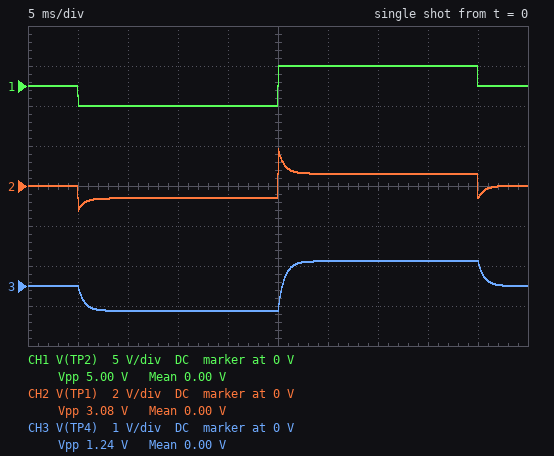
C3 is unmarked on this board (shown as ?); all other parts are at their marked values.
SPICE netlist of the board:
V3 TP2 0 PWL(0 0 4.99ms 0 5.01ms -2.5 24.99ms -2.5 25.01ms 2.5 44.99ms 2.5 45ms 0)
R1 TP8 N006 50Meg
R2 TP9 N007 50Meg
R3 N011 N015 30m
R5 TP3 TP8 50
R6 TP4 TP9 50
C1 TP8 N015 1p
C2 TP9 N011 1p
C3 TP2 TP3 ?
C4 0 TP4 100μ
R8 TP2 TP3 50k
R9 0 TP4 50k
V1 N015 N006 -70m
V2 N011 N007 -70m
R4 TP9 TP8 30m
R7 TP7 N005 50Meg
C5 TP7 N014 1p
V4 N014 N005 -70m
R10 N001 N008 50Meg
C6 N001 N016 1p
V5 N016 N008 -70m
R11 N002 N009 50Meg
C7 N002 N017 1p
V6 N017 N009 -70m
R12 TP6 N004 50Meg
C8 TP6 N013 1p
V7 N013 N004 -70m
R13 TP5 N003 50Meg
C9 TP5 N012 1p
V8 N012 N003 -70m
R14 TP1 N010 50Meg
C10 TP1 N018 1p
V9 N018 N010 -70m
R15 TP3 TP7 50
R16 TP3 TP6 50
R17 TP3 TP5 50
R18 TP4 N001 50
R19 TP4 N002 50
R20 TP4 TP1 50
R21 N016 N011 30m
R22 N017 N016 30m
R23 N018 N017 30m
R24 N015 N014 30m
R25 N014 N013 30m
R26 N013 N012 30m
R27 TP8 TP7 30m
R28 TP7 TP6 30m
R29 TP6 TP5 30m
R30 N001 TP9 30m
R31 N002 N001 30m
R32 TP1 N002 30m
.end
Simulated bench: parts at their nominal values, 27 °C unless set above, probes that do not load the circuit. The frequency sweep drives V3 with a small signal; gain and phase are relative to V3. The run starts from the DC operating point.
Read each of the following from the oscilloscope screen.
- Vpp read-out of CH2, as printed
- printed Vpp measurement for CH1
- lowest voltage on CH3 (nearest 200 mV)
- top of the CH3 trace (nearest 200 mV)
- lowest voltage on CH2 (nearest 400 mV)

3.08 V
5.00 V
-600 mV
600 mV
-1.2 V
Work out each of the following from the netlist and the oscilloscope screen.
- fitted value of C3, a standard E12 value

33 µF
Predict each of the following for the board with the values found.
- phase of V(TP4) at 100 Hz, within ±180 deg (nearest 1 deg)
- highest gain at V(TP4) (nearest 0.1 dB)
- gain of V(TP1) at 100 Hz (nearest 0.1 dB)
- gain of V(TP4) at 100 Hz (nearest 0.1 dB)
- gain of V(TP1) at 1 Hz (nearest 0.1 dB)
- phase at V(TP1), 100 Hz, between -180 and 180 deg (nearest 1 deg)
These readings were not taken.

-21 deg
-6.0 dB
-10.6 dB
-12.7 dB
-12.1 dB
17 deg
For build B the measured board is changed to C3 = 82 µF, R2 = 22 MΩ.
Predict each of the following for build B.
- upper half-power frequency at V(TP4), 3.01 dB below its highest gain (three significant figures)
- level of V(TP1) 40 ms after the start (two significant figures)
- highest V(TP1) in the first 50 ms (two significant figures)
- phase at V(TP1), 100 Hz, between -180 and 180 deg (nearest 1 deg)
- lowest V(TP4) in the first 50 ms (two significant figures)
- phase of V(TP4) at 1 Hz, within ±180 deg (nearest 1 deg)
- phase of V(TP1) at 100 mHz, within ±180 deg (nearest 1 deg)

111 Hz
1.1 V
1.4 V
3 deg
-1.1 V
-1 deg
-2 deg
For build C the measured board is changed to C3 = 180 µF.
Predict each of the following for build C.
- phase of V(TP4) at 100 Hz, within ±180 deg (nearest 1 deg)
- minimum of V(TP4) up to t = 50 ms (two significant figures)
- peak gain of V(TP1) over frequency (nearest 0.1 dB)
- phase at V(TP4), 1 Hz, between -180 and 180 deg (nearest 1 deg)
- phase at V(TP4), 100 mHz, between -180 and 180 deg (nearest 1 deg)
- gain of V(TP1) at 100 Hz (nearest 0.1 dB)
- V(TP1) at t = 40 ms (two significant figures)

-45 deg
-1.6 V
-3.8 dB
0 deg
3 deg
-4.8 dB
1.6 V
